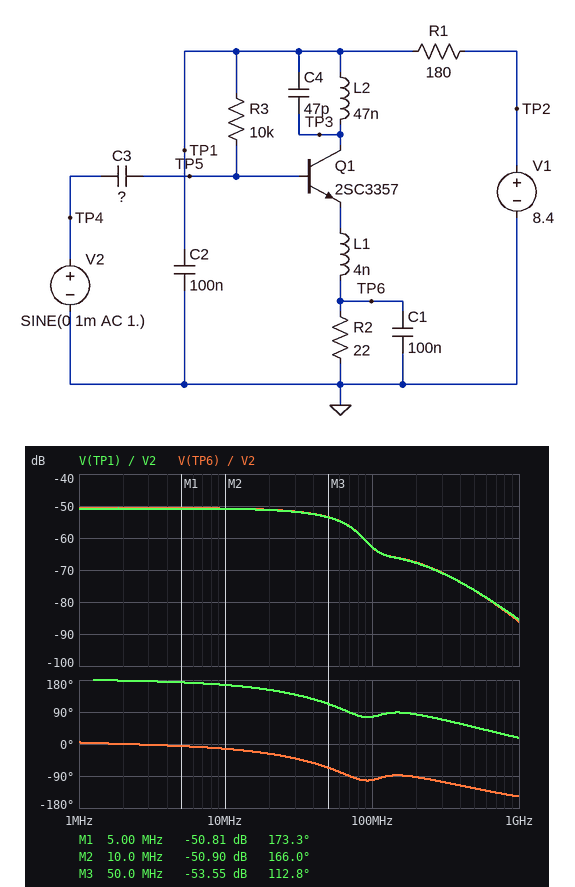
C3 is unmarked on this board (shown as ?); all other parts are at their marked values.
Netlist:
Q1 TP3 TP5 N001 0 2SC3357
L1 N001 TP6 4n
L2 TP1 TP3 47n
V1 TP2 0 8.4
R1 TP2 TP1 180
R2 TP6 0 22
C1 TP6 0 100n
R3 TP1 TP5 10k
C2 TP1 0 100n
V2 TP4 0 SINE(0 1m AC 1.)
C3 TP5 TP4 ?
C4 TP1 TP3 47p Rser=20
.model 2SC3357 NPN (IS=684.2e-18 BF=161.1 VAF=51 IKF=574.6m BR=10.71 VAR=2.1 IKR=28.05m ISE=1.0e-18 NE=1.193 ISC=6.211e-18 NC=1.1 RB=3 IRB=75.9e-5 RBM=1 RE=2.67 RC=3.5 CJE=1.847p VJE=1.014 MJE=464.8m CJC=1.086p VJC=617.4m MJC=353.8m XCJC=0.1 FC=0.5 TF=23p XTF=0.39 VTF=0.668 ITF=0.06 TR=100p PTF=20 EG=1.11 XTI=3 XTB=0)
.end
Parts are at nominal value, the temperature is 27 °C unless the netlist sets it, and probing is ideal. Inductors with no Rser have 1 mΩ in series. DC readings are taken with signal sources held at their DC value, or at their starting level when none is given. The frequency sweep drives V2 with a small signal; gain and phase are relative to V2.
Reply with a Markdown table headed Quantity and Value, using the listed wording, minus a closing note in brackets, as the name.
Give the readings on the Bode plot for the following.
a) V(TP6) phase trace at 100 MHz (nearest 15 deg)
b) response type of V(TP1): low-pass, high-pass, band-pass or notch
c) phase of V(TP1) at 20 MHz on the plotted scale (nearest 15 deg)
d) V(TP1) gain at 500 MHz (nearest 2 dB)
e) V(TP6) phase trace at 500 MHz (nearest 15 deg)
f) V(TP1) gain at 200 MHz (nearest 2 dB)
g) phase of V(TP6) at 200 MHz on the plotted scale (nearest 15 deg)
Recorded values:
| Quantity | Value |
|---|---|
| V(TP6) phase trace at 100 MHz | -105 deg |
| response type of V(TP1): low-pass, high-pass, band-pass or notch | low-pass |
| phase of V(TP1) at 20 MHz on the plotted scale | 150 deg |
| V(TP1) gain at 500 MHz | -76 dB |
| V(TP6) phase trace at 500 MHz | -120 deg |
| V(TP1) gain at 200 MHz | -68 dB |
| phase of V(TP6) at 200 MHz on the plotted scale | -90 deg |
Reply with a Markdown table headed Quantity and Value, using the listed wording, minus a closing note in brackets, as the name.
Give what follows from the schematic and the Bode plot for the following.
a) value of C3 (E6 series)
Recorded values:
| Quantity | Value |
|---|---|
| value of C3 | 3.3 pF |
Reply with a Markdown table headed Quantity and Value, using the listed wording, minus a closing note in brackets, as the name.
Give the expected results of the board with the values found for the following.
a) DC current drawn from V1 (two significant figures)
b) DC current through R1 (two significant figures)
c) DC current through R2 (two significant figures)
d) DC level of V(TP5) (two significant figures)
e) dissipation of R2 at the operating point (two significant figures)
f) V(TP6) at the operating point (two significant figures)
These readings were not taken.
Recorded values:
| Quantity | Value |
|---|---|
| DC current drawn from V1 | 25 mA |
| DC current through R1 | 25 mA |
| DC current through R2 | 25 mA |
| DC level of V(TP5) | 1.4 V |
| dissipation of R2 at the operating point | 14 mW |
| V(TP6) at the operating point | 550 mV |
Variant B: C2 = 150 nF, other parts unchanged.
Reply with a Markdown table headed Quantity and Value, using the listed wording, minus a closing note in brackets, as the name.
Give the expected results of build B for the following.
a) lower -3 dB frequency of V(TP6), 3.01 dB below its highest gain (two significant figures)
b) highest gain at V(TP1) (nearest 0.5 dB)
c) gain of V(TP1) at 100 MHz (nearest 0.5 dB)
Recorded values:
| Quantity | Value |
|---|---|
| lower -3 dB frequency of V(TP6), 3.01 dB below its highest gain | 91 kHz |
| highest gain at V(TP1) | -54.5 dB |
| gain of V(TP1) at 100 MHz | -66.5 dB |
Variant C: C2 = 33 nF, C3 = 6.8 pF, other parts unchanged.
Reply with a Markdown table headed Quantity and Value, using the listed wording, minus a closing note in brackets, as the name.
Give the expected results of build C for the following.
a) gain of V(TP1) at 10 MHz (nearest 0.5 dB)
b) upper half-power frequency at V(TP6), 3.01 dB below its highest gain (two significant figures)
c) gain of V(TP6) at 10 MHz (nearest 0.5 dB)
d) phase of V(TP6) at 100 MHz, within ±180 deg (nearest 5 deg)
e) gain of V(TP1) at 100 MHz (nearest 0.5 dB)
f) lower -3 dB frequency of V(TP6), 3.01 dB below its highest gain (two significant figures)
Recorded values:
| Quantity | Value |
|---|---|
| gain of V(TP1) at 10 MHz | -35.0 dB |
| upper half-power frequency at V(TP6), 3.01 dB below its highest gain | 39 MHz |
| gain of V(TP6) at 10 MHz | -44.5 dB |
| phase of V(TP6) at 100 MHz, within ±180 deg | -105 deg |
| gain of V(TP1) at 100 MHz | -48.5 dB |
| lower -3 dB frequency of V(TP6), 3.01 dB below its highest gain | 120 kHz |
